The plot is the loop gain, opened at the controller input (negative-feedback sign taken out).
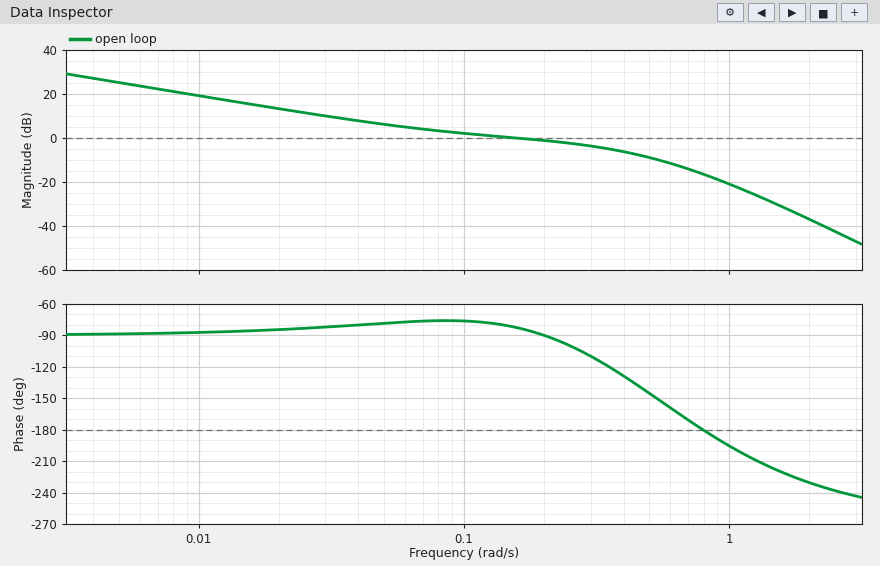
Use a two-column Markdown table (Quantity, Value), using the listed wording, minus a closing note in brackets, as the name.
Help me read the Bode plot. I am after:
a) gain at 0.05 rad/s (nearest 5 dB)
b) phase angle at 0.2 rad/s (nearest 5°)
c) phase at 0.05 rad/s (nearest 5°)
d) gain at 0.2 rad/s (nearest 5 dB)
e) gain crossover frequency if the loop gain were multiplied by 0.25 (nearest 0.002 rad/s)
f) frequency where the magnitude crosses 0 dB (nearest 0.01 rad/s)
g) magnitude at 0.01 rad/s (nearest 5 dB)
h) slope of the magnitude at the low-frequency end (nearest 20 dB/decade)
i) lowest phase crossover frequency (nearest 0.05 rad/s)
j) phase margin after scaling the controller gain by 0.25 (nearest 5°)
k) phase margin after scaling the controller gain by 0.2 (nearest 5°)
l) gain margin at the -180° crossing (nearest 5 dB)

| Quantity | Value |
|---|---|
| gain at 0.05 rad/s | 5 dB |
| phase angle at 0.2 rad/s | -90° |
| phase at 0.05 rad/s | -80° |
| gain at 0.2 rad/s | 0 dB |
| gain crossover frequency if the loop gain were multiplied by 0.25 | 0.024 rad/s |
| frequency where the magnitude crosses 0 dB | 0.16 rad/s |
| magnitude at 0.01 rad/s | 20 dB |
| slope of the magnitude at the low-frequency end | -20 dB/decade |
| lowest phase crossover frequency | 0.80 rad/s |
| phase margin after scaling the controller gain by 0.25 | 95° |
| phase margin after scaling the controller gain by 0.2 | 95° |
| gain margin at the -180° crossing | 15 dB |
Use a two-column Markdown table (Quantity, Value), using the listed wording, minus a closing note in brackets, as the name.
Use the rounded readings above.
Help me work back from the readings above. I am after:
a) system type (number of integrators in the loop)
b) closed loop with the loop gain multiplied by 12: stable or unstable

| Quantity | Value |
|---|---|
| system type | 1 |
| closed loop with the loop gain multiplied by 12: stable or unstable | unstable |
